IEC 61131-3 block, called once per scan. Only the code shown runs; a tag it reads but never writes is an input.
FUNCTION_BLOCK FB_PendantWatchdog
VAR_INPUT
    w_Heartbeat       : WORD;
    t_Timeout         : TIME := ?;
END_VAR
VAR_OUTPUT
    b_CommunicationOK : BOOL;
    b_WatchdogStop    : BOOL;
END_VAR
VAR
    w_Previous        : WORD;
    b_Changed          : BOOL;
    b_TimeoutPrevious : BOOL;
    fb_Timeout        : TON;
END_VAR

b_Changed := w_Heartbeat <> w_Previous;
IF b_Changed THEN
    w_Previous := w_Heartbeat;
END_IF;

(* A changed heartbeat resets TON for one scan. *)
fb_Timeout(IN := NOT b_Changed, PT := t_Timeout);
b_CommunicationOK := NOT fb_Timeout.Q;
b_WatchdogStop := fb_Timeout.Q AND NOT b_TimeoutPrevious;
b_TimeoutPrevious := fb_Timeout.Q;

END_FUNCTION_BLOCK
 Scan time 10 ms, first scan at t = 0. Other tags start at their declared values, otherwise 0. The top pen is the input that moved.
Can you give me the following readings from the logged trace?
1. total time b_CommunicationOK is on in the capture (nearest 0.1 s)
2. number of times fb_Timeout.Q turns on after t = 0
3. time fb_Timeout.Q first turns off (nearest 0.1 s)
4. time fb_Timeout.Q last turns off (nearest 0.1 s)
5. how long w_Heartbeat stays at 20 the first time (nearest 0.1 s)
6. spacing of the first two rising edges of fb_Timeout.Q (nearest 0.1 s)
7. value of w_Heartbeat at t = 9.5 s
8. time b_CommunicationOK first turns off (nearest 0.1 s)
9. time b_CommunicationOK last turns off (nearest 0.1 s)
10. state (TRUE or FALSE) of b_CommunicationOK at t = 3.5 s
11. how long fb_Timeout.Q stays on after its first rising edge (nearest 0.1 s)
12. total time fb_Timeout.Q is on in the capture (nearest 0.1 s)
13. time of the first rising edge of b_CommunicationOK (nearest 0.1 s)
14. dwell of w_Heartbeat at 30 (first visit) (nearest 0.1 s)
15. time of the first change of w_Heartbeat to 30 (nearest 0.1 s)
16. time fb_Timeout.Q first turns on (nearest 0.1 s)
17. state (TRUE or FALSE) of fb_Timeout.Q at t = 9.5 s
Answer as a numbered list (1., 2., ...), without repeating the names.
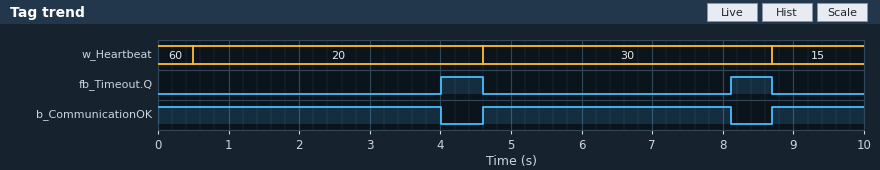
1. 8.8 s
2. 2
3. 4.6 s
4. 8.7 s
5. 4.1 s
6. 4.1 s
7. 15
8. 4.0 s
9. 8.1 s
10. TRUE
11. 0.6 s
12. 1.2 s
13. 4.6 s
14. 4.1 s
15. 4.6 s
16. 4.0 s
17. FALSE
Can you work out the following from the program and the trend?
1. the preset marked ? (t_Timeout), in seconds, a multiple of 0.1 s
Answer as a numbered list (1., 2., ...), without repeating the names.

1. 3.5 s
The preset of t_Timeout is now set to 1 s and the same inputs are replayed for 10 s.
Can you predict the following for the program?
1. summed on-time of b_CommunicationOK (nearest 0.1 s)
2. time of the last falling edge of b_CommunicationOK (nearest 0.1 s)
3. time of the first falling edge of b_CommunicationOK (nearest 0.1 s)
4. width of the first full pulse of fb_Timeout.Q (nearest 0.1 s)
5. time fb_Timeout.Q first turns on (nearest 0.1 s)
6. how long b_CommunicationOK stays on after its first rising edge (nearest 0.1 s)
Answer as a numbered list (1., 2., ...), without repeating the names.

1. 3.5 s
2. 9.7 s
3. 1.5 s
4. 3.1 s
5. 1.5 s
6. 1.0 s
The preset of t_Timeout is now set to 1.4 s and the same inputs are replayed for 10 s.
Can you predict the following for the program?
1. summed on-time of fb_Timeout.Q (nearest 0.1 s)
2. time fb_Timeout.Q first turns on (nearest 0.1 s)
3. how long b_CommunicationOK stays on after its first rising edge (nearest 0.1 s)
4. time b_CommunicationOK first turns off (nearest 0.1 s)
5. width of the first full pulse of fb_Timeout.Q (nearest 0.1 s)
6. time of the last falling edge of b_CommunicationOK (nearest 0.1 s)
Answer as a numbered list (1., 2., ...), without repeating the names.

1. 5.4 s
2. 1.9 s
3. 1.4 s
4. 1.9 s
5. 2.7 s
6. 6.0 s
